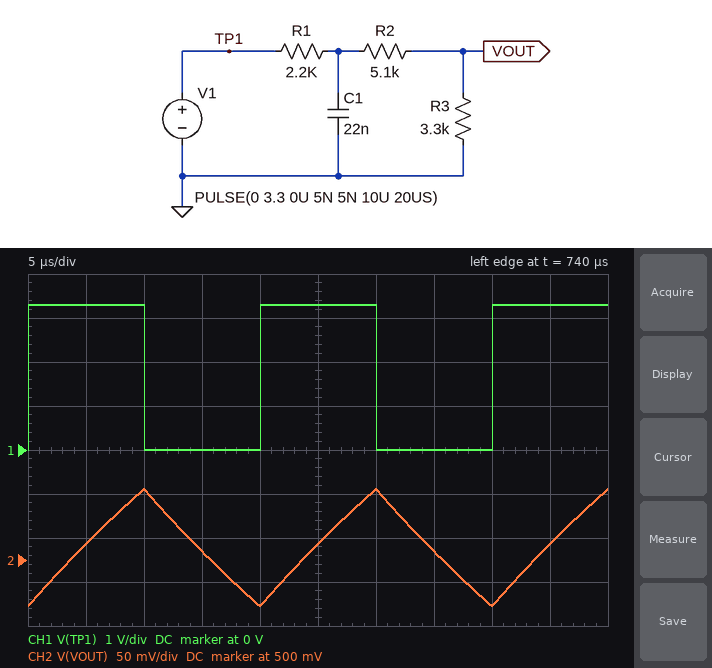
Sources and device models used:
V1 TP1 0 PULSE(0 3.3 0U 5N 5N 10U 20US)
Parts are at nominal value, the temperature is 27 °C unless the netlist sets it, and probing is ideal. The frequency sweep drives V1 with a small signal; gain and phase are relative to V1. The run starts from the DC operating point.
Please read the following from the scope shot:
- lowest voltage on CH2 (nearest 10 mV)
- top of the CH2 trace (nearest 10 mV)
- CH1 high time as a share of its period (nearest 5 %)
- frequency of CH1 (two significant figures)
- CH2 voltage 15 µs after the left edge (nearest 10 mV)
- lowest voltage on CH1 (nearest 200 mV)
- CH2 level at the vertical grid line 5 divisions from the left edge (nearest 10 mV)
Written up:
450 mV
580 mV
50 %
50 kHz
510 mV
0 V
520 mV
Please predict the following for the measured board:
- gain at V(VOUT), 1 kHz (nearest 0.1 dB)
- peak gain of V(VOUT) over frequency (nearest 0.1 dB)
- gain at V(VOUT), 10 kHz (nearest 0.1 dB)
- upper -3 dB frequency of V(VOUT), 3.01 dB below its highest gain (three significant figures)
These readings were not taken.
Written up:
-10.4 dB
-10.1 dB
-18.5 dB
4.15 kHz
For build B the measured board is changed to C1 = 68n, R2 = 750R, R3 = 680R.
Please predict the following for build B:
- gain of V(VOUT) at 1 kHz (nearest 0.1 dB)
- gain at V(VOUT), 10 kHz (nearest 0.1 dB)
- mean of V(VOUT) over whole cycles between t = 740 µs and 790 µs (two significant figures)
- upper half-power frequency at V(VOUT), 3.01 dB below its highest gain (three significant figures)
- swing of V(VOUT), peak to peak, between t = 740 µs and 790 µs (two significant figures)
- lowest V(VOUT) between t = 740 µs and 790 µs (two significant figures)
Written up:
-15.1 dB
-26.2 dB
310 mV
2.70 kHz
52 mV
280 mV
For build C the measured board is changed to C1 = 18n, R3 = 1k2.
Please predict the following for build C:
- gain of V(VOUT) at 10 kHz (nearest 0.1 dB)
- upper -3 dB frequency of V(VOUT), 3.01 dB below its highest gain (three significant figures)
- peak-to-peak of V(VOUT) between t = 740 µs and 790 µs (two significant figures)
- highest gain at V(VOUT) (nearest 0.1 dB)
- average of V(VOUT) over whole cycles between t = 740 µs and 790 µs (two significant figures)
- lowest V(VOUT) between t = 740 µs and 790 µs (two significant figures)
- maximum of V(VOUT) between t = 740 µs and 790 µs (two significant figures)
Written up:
-23.4 dB
5.42 kHz
79 mV
-17.0 dB
230 mV
190 mV
270 mV
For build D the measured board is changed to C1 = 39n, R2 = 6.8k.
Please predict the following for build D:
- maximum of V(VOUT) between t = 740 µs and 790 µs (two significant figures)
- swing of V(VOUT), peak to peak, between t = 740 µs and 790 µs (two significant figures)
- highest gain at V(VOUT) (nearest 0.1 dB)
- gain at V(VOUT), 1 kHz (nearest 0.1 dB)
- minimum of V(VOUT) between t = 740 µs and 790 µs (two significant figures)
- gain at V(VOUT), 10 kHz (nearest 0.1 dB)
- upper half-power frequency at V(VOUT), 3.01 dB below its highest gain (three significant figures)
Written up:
470 mV
63 mV
-11.4 dB
-12.2 dB
410 mV
-24.6 dB
2.26 kHz
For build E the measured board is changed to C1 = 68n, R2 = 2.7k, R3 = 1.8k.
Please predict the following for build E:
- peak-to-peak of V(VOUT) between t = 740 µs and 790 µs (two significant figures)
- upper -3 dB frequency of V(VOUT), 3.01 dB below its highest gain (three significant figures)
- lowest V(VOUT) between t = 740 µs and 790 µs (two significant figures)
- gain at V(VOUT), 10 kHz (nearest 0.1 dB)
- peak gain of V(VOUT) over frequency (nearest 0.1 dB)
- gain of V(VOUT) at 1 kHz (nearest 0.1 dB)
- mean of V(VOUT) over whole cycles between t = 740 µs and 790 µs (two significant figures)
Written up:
44 mV
1.58 kHz
420 mV
-27.5 dB
-11.4 dB
-12.9 dB
440 mV
